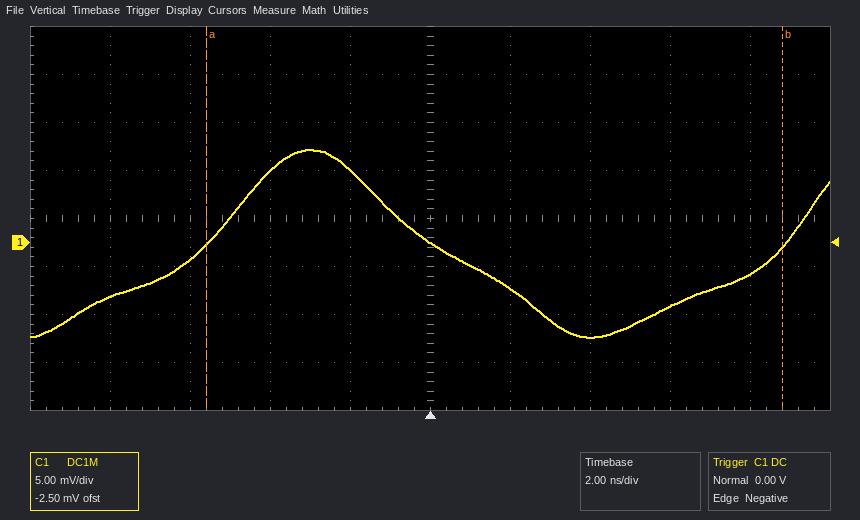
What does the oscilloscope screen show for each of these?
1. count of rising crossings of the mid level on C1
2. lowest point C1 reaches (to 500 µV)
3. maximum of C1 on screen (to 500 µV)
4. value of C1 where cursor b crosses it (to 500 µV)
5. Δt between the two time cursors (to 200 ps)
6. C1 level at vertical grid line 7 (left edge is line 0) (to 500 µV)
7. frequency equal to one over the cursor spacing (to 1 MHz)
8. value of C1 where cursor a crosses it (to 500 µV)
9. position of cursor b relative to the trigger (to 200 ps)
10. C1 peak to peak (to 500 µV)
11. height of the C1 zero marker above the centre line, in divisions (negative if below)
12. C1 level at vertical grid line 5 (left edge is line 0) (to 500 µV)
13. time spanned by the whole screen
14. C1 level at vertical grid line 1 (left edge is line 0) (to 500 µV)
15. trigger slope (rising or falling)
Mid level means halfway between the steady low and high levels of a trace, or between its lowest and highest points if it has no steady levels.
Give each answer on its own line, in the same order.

2
-10.0 mV
9.5 mV
-500 µV
14.4 ns
-10.0 mV
69 MHz
0.0 mV
+8.8 ns
19.5 mV
-0.5 div
0.0 mV
20 ns
-5.5 mV
falling
